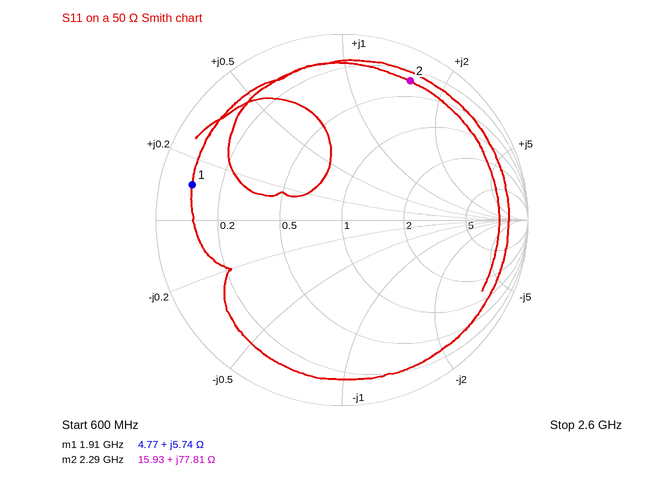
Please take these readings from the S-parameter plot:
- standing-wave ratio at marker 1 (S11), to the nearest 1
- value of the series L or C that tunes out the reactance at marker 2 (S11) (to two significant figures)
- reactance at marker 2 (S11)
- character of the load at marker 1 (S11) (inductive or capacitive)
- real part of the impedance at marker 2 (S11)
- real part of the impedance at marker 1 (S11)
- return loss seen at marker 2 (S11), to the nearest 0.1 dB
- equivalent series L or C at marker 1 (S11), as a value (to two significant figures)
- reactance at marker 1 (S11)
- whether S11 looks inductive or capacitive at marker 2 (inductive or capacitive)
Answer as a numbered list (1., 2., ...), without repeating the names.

1. 11
2. 890 fF
3. +77.81 Ω
4. inductive
5. 15.93 Ω
6. 4.77 Ω
7. 1.6 dB
8. 480 pH
9. +5.74 Ω
10. inductive
